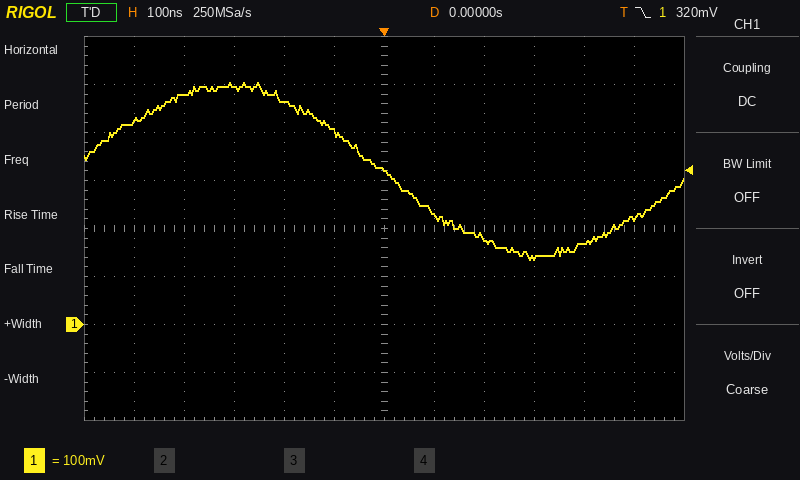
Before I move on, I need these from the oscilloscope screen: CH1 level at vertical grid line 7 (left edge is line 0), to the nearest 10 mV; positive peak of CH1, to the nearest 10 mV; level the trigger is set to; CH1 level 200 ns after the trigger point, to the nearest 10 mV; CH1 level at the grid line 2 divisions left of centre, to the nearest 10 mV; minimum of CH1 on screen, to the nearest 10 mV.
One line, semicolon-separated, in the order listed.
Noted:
230 mV; 500 mV; 320 mV; 180 mV; 460 mV; 140 mV
